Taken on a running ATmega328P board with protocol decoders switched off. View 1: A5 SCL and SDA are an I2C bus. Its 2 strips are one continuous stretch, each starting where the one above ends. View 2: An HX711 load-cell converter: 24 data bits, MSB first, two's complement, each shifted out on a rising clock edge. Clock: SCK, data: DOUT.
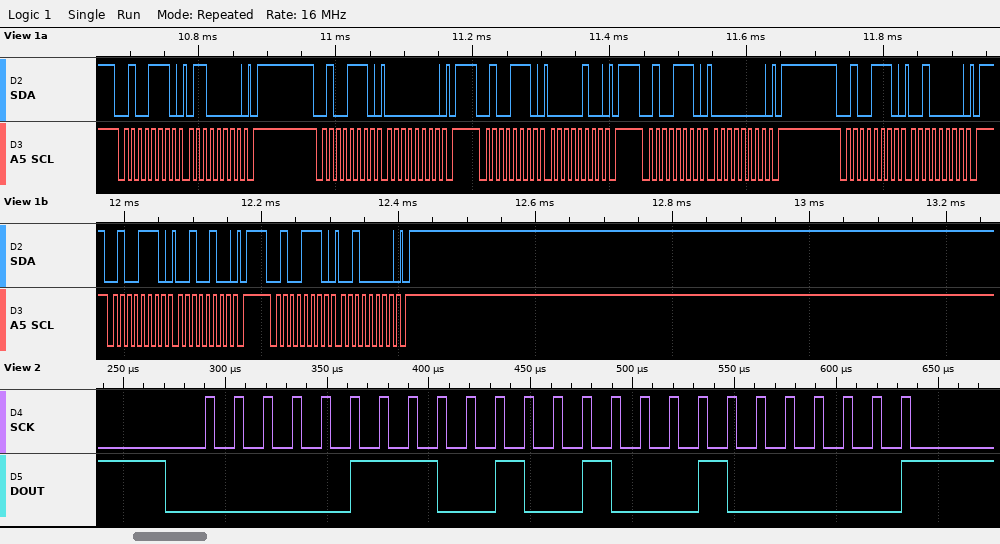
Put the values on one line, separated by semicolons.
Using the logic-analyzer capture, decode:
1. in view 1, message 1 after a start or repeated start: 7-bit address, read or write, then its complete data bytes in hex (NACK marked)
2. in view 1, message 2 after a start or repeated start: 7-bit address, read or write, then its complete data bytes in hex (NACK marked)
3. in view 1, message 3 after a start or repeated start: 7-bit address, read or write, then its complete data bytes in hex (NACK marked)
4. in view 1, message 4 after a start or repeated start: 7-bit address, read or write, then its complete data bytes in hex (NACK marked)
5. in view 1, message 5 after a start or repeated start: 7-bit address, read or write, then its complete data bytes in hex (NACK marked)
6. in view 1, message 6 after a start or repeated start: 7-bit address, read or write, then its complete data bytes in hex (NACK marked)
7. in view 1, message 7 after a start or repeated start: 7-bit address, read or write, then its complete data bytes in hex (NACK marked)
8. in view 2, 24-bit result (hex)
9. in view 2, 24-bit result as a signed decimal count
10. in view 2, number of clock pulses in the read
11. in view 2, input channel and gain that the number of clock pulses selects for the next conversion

0x27 write: 60; 0x27 write: 00; 0x27 write: 04; 0x27 write: 00; 0x27 write: 20; 0x27 write: 24; 0x27 write: 20; 0x072440; 468032; 25; channel A, gain 128
